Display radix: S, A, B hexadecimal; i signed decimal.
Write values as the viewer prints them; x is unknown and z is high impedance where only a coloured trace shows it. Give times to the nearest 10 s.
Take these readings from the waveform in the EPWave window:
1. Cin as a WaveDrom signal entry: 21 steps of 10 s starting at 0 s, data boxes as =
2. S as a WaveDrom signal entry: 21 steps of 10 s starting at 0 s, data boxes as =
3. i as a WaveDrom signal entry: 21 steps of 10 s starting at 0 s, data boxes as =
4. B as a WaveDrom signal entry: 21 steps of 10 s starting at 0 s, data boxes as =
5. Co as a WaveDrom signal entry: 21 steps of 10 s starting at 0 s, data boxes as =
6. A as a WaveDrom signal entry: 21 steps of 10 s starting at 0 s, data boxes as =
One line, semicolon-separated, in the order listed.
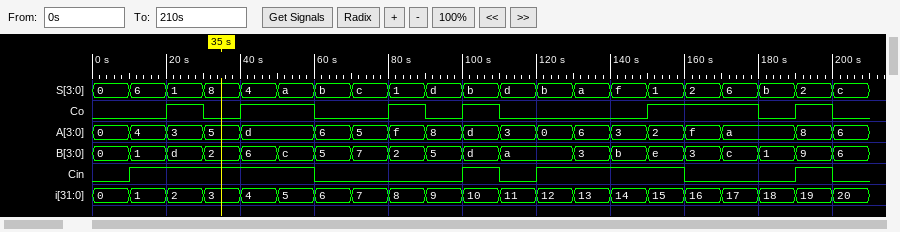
{name: 'Cin', wave: '01....0...101...0..10'}; {name: 'S', wave: '=====================', data: '0 6 1 8 4 a b c 1 d b d b a f 1 2 6 b 2 c'}; {name: 'i', wave: '=====================', data: '0 1 2 3 4 5 6 7 8 9 10 11 12 13 14 15 16 17 18 19 20'}; {name: 'B', wave: '============.========', data: '0 1 d 2 6 c 5 7 2 5 d a 3 b e 3 c 1 9 6'}; {name: 'Co', wave: '0.101.0.1010...1..010'}; {name: 'A', wave: '=====.============.==', data: '0 4 3 5 d 6 5 f 8 d 3 0 6 3 2 f a 8 6'}
